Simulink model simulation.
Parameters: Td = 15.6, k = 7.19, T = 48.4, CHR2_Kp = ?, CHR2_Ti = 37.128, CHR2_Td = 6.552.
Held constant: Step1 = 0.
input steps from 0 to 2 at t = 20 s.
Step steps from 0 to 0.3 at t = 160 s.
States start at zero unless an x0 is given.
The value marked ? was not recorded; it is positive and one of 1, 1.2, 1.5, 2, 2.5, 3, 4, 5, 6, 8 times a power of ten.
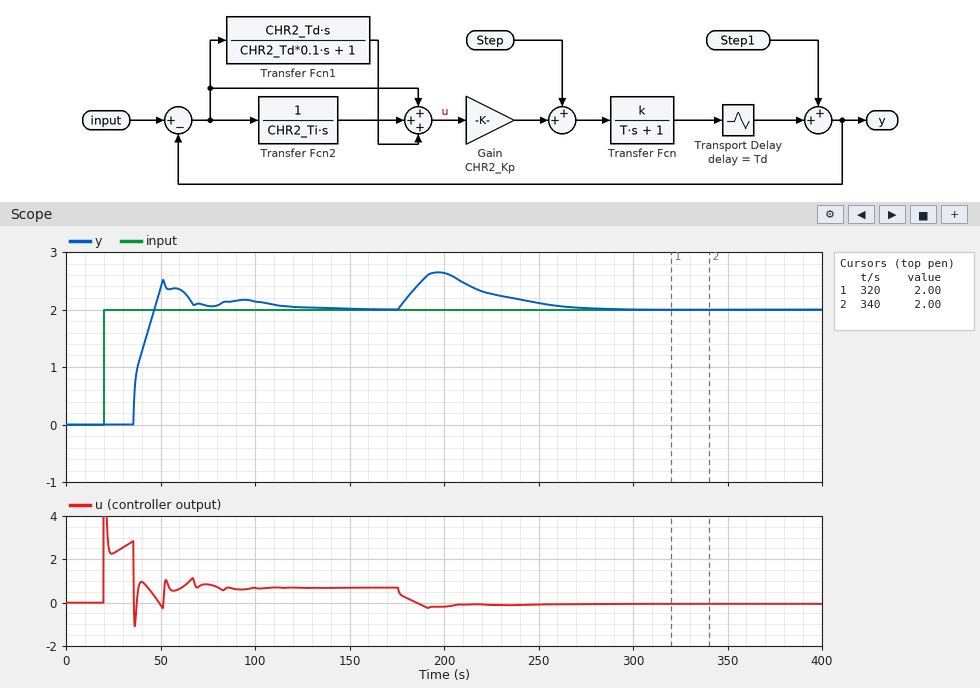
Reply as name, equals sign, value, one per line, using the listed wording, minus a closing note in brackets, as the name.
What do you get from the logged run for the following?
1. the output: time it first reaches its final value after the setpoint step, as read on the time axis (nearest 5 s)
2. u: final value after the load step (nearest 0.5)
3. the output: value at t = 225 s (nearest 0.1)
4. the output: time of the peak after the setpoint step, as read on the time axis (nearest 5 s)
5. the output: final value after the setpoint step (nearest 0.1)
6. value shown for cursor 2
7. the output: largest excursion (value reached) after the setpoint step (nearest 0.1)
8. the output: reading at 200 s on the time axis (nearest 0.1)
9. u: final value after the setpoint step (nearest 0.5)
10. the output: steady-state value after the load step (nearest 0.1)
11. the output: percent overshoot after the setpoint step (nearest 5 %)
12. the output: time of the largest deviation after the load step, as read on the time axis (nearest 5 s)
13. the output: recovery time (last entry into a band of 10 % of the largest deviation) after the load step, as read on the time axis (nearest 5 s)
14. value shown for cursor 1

the output: time it first reaches its final value after the setpoint step, as read on the time axis = 45 s
u: final value after the load step = 0.0
the output: value at t = 225 s = 2.3
the output: time of the peak after the setpoint step, as read on the time axis = 50 s
the output: final value after the setpoint step = 2.0
value shown for cursor 2 = 2.00
the output: largest excursion (value reached) after the setpoint step = 2.5
the output: reading at 200 s on the time axis = 2.6
u: final value after the setpoint step = 0.5
the output: steady-state value after the load step = 2.0
the output: percent overshoot after the setpoint step = 25 %
the output: time of the largest deviation after the load step, as read on the time axis = 195 s
the output: recovery time (last entry into a band of 10 % of the largest deviation) after the load step, as read on the time axis = 260 s
value shown for cursor 1 = 2.00
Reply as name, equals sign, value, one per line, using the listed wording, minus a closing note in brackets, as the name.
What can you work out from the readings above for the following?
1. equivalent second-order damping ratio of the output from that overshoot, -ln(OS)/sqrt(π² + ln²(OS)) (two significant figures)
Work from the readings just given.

equivalent second-order damping ratio of the output from that overshoot, -ln(OS)/sqrt(π² + ln²(OS)) = 0.40
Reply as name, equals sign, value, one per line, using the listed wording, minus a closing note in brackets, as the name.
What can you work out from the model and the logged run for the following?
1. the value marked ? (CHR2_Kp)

the value marked ? = 0.4
